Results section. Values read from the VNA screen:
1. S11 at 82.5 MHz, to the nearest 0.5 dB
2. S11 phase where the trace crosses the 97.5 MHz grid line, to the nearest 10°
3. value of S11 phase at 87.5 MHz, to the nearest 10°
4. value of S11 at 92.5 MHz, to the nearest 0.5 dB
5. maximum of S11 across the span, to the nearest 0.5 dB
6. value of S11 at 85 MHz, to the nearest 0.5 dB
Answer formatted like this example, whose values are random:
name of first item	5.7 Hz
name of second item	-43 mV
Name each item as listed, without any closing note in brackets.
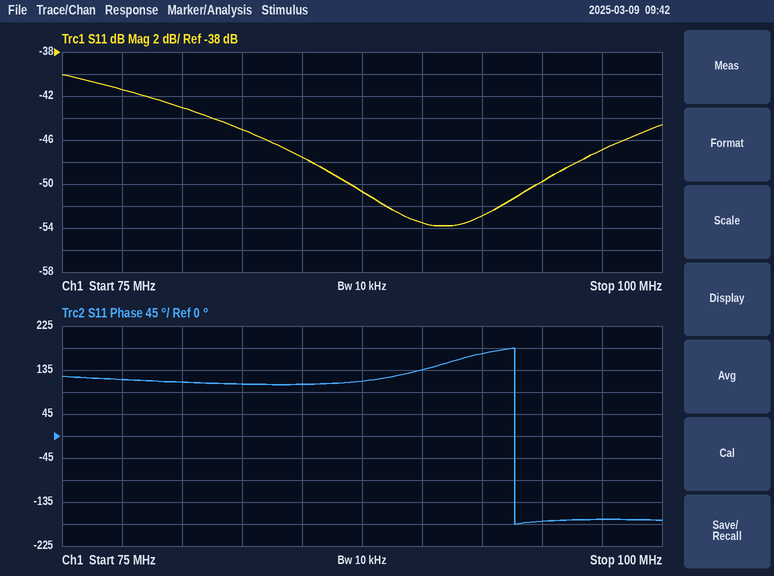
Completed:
S11 at 82.5 MHz, to the nearest 0.5 dB	-45.0 dB
S11 phase where the trace crosses the 97.5 MHz grid line, to the nearest 10°	-170°
value of S11 phase at 87.5 MHz, to the nearest 10°	110°
value of S11 at 92.5 MHz, to the nearest 0.5 dB	-53.0 dB
maximum of S11 across the span, to the nearest 0.5 dB	-40.0 dB
value of S11 at 85 MHz, to the nearest 0.5 dB	-47.5 dB
